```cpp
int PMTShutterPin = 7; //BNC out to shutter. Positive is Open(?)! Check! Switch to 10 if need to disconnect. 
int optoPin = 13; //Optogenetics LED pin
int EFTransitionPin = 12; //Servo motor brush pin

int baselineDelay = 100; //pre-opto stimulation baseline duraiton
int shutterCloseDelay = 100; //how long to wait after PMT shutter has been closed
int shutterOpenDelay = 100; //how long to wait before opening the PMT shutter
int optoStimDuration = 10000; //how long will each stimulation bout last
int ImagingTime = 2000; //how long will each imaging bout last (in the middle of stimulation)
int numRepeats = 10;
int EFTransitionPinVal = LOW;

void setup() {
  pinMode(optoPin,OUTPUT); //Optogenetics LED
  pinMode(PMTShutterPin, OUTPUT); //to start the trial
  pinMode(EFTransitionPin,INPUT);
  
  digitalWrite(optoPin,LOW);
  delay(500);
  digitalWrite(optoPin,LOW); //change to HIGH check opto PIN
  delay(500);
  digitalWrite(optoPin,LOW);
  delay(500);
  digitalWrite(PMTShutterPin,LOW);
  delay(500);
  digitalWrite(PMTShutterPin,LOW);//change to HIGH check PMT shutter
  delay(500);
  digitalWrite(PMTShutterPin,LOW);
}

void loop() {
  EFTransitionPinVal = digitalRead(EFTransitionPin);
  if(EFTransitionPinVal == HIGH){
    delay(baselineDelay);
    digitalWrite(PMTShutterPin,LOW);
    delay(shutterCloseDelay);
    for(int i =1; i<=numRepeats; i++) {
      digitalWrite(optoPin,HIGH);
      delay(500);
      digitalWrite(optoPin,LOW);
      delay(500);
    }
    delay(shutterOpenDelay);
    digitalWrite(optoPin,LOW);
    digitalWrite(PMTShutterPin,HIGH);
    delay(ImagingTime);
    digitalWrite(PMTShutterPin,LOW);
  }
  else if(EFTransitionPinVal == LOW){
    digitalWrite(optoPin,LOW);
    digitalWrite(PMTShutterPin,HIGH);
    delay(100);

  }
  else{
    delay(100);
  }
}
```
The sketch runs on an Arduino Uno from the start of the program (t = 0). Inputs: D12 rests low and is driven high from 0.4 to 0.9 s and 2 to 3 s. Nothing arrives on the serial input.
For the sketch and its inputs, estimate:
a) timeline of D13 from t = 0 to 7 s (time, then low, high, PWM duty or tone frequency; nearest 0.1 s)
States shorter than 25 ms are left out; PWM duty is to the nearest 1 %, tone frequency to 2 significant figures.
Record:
0 s low; 2.7 s high; 3.2 s low; 3.7 s high; 4.2 s low; 4.7 s high; 5.2 s low; 5.7 s high; 6.2 s low; 6.7 s high
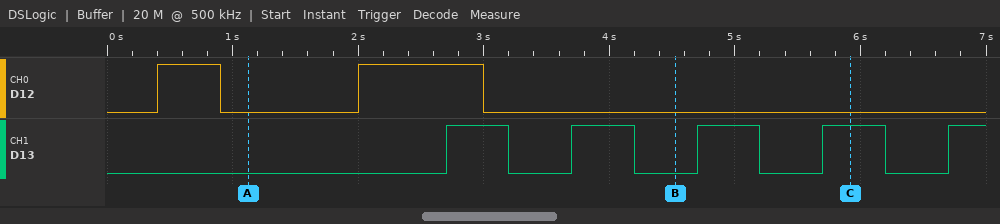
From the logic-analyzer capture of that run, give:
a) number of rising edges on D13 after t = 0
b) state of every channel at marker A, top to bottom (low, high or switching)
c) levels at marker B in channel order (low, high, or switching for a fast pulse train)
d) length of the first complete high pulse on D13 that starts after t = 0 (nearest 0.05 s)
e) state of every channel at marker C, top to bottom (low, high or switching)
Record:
5
D12 low, D13 low
D12 low, D13 low
0.50 s
D12 low, D13 high
